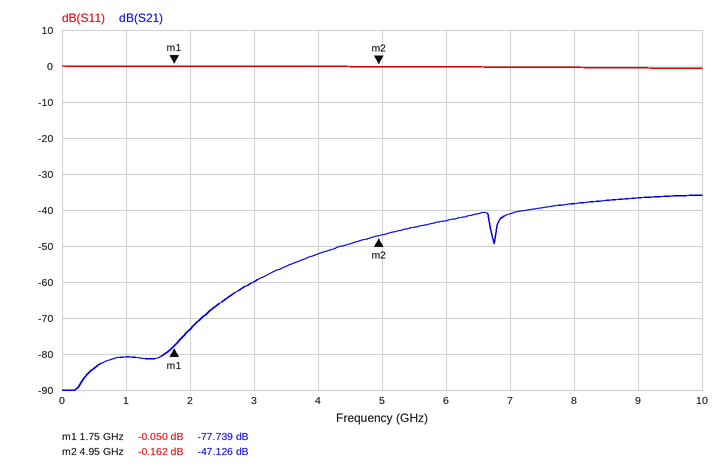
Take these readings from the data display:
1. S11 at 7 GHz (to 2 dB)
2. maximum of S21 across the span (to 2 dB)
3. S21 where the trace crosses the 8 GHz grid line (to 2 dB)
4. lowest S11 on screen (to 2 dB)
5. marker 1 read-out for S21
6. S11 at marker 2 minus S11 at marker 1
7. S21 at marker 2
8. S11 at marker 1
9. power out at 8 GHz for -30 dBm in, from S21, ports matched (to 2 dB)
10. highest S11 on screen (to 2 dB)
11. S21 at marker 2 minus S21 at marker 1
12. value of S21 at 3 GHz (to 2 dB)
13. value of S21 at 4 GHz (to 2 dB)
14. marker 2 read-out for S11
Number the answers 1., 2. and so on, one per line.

1. 0 dB
2. -36 dB
3. -38 dB
4. 0 dB
5. -77.739 dB
6. -0.112 dB
7. -47.126 dB
8. -0.050 dB
9. -68 dBm
10. 0 dB
11. 30.613 dB
12. -60 dB
13. -52 dB
14. -0.162 dB
